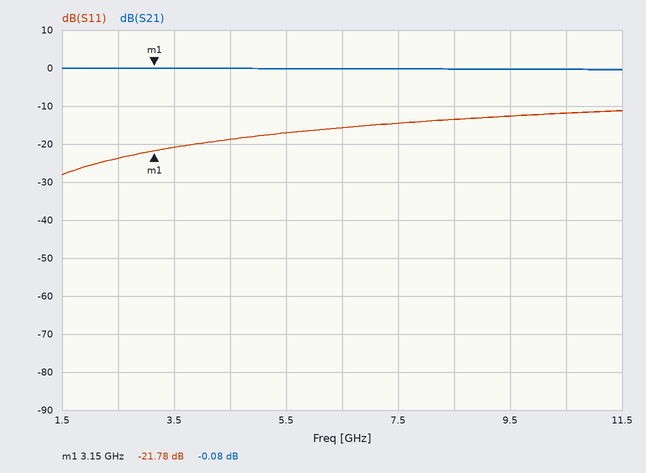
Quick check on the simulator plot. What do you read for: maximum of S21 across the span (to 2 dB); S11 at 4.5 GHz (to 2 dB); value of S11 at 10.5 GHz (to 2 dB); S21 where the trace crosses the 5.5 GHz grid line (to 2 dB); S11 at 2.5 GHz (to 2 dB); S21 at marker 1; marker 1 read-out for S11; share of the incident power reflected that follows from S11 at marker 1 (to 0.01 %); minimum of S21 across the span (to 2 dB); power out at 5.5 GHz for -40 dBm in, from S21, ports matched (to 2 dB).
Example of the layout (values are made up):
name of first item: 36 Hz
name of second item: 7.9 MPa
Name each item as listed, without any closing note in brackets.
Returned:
maximum of S21 across the span: 0 dB
S11 at 4.5 GHz: -18 dB
value of S11 at 10.5 GHz: -12 dB
S21 where the trace crosses the 5.5 GHz grid line: 0 dB
S11 at 2.5 GHz: -24 dB
S21 at marker 1: -0.08 dB
marker 1 read-out for S11: -21.78 dB
share of the incident power reflected that follows from S11 at marker 1: 0.66 %
minimum of S21 across the span: 0 dB
power out at 5.5 GHz for -40 dBm in, from S21, ports matched: -40 dBm
